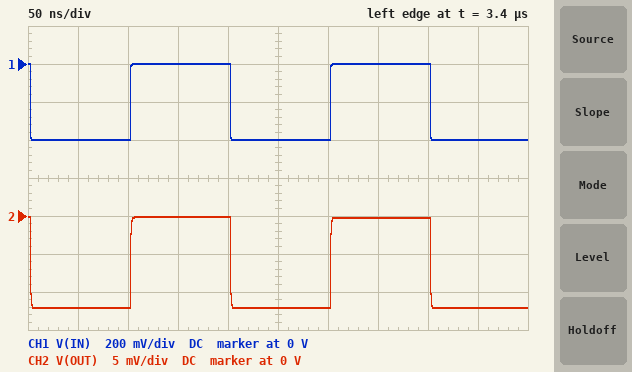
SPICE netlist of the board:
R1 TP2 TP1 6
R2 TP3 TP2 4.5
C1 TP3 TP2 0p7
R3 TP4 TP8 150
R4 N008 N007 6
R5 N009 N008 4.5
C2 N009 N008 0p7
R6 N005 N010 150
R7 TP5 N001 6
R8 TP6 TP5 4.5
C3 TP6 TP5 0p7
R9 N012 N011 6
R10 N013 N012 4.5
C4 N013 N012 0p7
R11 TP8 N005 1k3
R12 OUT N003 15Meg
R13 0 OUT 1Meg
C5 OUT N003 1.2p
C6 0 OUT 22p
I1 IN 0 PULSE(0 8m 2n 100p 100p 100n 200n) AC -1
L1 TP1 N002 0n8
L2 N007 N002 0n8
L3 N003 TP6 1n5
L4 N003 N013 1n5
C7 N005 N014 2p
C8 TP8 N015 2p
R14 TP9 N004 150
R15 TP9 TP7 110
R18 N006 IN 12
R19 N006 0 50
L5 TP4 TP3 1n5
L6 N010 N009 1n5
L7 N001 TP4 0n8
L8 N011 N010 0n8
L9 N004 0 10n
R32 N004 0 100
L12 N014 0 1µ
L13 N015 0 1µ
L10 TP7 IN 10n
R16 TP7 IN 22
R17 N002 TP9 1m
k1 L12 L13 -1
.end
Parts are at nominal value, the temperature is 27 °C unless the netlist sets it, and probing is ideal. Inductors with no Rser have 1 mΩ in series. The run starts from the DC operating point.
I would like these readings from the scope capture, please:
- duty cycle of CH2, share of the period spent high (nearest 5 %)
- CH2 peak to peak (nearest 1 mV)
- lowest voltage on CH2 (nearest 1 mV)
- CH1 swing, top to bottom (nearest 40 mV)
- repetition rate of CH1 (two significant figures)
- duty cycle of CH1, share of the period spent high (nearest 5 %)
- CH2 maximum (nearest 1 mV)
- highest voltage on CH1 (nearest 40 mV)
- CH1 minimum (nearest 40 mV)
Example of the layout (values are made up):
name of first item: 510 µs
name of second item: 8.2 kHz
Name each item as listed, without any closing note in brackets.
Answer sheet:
duty cycle of CH2, share of the period spent high: 50 %
CH2 peak to peak: 12 mV
lowest voltage on CH2: -12 mV
CH1 swing, top to bottom: 400 mV
repetition rate of CH1: 5.0 MHz
duty cycle of CH1, share of the period spent high: 50 %
CH2 maximum: 0 V
highest voltage on CH1: 0 V
CH1 minimum: -400 mV
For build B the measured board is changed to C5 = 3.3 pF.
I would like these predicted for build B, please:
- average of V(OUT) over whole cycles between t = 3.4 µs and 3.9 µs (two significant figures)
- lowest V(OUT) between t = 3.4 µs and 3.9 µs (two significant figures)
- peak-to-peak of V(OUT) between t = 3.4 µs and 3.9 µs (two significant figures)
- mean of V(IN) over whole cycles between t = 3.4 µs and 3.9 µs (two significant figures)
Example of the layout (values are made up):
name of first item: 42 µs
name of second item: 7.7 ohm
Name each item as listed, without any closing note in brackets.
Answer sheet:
average of V(OUT) over whole cycles between t = 3.4 µs and 3.9 µs: -14 mV
lowest V(OUT) between t = 3.4 µs and 3.9 µs: -29 mV
peak-to-peak of V(OUT) between t = 3.4 µs and 3.9 µs: 30 mV
mean of V(IN) over whole cycles between t = 3.4 µs and 3.9 µs: -200 mV
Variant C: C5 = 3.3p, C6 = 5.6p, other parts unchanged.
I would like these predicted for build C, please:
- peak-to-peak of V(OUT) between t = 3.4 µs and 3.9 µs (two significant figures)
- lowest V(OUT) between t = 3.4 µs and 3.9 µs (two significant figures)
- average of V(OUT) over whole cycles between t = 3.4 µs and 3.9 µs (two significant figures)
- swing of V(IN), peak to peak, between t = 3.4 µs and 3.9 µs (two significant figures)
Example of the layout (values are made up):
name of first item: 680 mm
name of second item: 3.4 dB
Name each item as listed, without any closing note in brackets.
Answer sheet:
peak-to-peak of V(OUT) between t = 3.4 µs and 3.9 µs: 87 mV
lowest V(OUT) between t = 3.4 µs and 3.9 µs: -74 mV
average of V(OUT) over whole cycles between t = 3.4 µs and 3.9 µs: -30 mV
swing of V(IN), peak to peak, between t = 3.4 µs and 3.9 µs: 400 mV
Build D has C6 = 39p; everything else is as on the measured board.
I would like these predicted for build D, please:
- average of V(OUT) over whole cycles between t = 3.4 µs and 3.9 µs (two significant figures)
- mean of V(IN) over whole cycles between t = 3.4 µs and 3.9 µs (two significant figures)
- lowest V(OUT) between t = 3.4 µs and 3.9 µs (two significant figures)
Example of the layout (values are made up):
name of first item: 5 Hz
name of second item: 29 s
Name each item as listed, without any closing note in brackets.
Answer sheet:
average of V(OUT) over whole cycles between t = 3.4 µs and 3.9 µs: -3.8 mV
mean of V(IN) over whole cycles between t = 3.4 µs and 3.9 µs: -200 mV
lowest V(OUT) between t = 3.4 µs and 3.9 µs: -7.3 mV
